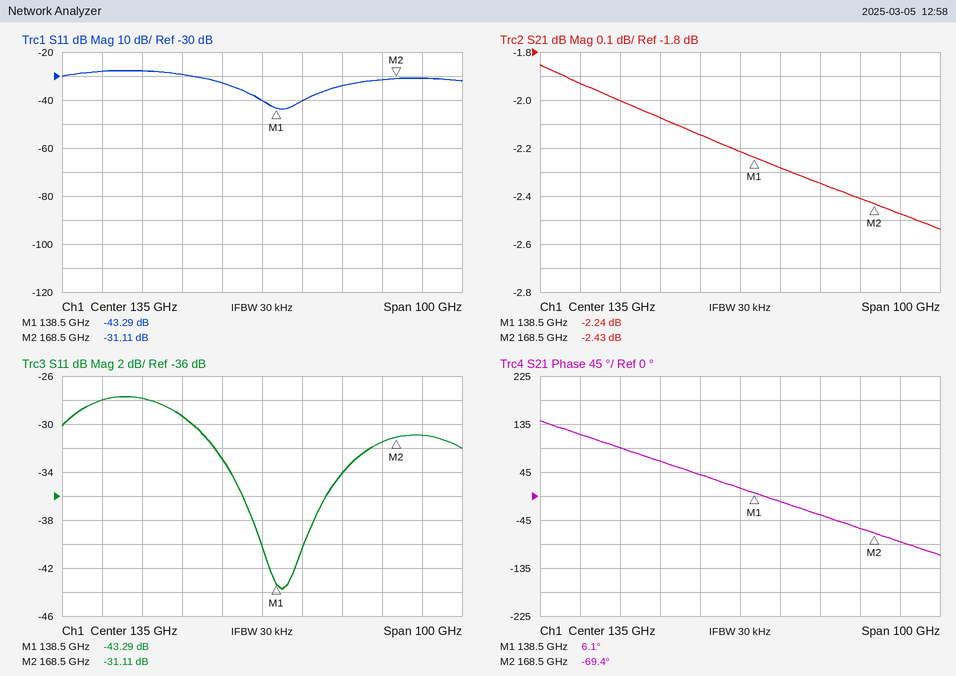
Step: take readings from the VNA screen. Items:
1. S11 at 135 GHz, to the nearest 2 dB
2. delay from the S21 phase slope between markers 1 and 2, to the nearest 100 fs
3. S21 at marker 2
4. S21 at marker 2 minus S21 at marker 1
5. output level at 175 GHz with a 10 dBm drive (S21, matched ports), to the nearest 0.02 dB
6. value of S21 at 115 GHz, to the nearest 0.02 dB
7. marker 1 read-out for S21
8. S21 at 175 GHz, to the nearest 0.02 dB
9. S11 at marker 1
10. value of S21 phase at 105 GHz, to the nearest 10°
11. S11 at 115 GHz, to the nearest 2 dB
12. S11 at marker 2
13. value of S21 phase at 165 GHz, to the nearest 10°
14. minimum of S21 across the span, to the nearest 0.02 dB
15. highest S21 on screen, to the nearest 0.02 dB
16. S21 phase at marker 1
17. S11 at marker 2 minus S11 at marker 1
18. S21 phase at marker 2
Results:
-40 dB
7.0 ps
-2.43 dB
-0.19 dB
7.52 dBm
-2.08 dB
-2.24 dB
-2.48 dB
-43.29 dB
90°
-30 dB
-31.11 dB
-60°
-2.54 dB
-1.86 dB
6.1°
12.18 dB
-69.4°
